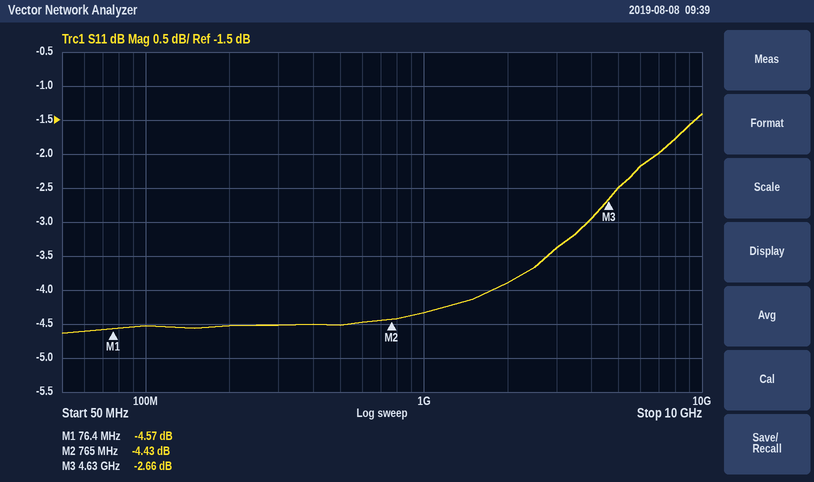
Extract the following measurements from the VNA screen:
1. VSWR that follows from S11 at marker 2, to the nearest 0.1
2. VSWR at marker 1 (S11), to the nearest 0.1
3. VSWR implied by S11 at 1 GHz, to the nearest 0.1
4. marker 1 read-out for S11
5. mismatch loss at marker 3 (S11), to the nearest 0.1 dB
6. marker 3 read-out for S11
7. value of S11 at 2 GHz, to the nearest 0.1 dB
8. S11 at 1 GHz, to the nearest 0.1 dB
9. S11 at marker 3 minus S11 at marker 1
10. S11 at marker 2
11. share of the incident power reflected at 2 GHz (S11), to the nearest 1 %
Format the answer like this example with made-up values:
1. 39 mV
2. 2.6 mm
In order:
1. 4.0
2. 3.9
3. 4.1
4. -4.57 dB
5. 3.4 dB
6. -2.66 dB
7. -3.9 dB
8. -4.3 dB
9. 1.91 dB
10. -4.43 dB
11. 41 %
